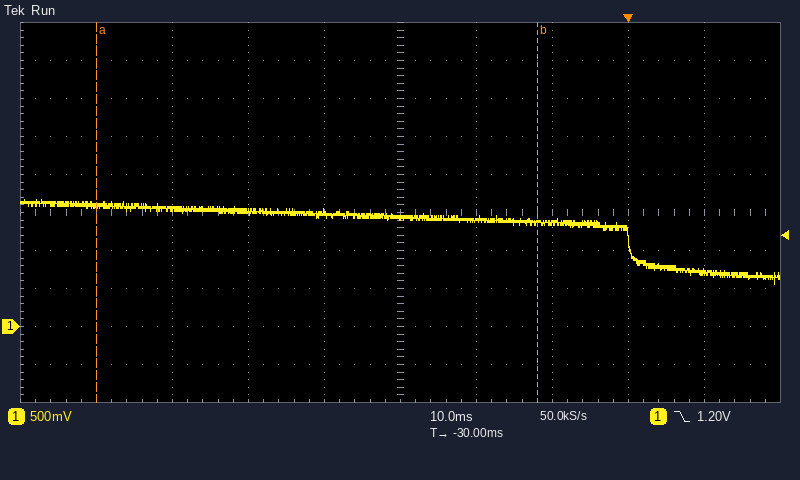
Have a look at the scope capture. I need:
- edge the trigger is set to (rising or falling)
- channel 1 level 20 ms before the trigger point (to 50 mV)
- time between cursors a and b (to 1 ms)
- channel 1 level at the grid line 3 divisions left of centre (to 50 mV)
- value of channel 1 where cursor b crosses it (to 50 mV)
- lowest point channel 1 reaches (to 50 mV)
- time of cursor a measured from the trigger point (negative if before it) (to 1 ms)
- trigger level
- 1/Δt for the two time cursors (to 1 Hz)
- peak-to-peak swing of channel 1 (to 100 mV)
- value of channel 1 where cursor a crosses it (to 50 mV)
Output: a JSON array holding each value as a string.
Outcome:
["falling", "1.40 V", "58 ms", "1.55 V", "1.35 V", "550 mV", "-70 ms", "1.20 V", "17 Hz", "1.10 V", "1.60 V"]
